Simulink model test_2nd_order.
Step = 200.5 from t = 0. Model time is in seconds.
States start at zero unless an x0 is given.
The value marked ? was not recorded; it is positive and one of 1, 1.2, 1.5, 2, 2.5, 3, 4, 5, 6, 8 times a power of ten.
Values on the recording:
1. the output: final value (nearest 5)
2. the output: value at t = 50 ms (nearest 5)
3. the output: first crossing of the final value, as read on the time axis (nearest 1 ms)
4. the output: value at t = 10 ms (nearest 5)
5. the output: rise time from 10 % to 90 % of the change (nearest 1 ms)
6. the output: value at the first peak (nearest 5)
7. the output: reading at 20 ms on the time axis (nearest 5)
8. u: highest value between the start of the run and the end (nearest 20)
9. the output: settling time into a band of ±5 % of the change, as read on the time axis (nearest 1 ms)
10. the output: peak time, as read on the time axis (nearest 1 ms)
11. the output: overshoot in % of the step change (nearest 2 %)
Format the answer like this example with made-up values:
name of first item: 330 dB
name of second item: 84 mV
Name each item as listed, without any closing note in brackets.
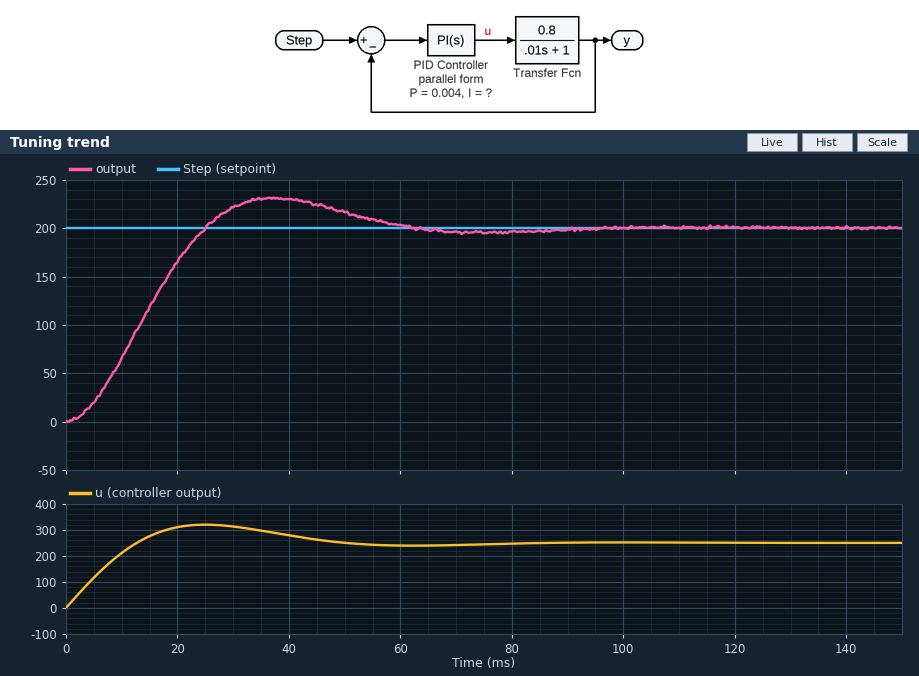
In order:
the output: final value: 200
the output: value at t = 50 ms: 215
the output: first crossing of the final value, as read on the time axis: 25 ms
the output: value at t = 10 ms: 65
the output: rise time from 10 % to 90 % of the change: 17 ms
the output: value at the first peak: 230
the output: reading at 20 ms on the time axis: 165
u: highest value between the start of the run and the end: 320
the output: settling time into a band of ±5 % of the change, as read on the time axis: 54 ms
the output: peak time, as read on the time axis: 37 ms
the output: overshoot in % of the step change: 16 %
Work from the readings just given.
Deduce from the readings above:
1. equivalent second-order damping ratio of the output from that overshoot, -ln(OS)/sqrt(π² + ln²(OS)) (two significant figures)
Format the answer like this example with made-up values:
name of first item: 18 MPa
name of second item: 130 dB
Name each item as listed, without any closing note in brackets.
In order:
equivalent second-order damping ratio of the output from that overshoot, -ln(OS)/sqrt(π² + ln²(OS)): 0.50
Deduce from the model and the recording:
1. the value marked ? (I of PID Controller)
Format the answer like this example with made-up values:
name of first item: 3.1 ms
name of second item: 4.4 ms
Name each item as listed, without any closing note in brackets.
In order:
the value marked ?: 120
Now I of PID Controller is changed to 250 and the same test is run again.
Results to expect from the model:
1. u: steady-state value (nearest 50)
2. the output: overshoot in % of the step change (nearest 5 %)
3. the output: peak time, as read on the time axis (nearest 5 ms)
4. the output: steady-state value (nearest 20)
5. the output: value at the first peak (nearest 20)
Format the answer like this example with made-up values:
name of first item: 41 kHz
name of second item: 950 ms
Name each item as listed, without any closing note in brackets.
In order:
u: steady-state value: 250
the output: overshoot in % of the step change: 30 %
the output: peak time, as read on the time axis: 25 ms
the output: steady-state value: 200
the output: value at the first peak: 260
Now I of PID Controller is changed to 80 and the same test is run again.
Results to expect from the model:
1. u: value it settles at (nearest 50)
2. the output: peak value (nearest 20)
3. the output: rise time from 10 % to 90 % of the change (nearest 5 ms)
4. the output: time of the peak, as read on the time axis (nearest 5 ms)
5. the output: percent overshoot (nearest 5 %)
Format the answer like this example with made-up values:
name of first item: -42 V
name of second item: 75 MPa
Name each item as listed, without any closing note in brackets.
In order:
u: value it settles at: 250
the output: peak value: 220
the output: rise time from 10 % to 90 % of the change: 25 ms
the output: time of the peak, as read on the time axis: 50 ms
the output: percent overshoot: 10 %
